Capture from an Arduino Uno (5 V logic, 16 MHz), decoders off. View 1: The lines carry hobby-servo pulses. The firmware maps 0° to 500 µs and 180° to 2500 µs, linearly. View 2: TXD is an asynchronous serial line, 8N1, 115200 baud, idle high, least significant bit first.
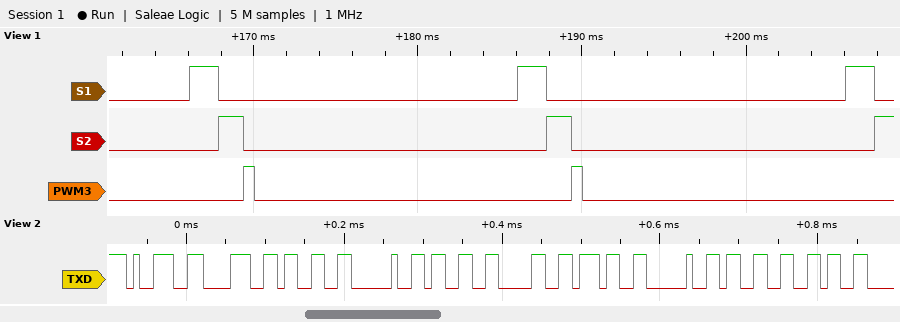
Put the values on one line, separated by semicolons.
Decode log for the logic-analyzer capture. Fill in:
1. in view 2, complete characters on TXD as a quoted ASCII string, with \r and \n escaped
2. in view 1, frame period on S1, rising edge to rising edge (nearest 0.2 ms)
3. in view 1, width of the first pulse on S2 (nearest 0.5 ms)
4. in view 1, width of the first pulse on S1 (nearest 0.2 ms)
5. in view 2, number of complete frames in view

"983 307 36"; 20.0 ms; 1.5 ms; 1.8 ms; 10
